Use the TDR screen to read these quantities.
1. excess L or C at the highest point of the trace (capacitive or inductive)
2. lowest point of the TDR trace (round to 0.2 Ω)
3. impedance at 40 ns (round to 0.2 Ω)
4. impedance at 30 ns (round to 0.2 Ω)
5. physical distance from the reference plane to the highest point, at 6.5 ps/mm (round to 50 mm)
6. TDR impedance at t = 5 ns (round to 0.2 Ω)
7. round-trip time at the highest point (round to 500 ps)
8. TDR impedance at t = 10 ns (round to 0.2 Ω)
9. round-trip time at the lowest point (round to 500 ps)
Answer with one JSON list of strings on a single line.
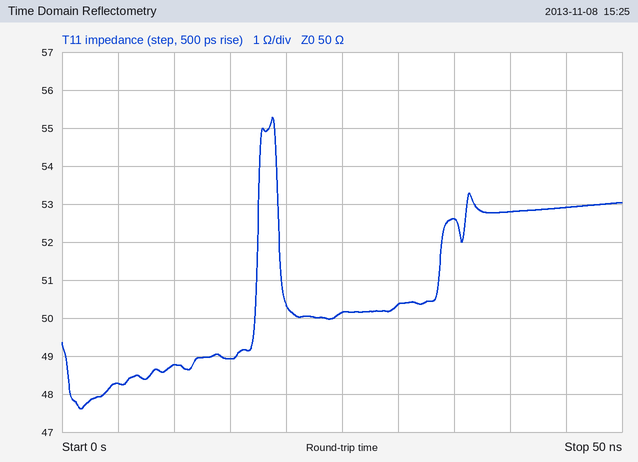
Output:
["inductive", "47.6 Ω", "52.8 Ω", "50.4 Ω", "1.45 m", "48.2 Ω", "19.0 ns", "48.8 Ω", "1.5 ns"]
